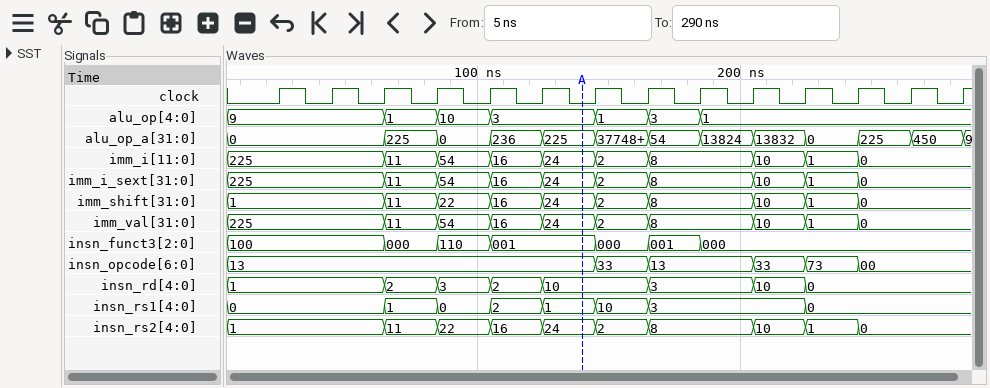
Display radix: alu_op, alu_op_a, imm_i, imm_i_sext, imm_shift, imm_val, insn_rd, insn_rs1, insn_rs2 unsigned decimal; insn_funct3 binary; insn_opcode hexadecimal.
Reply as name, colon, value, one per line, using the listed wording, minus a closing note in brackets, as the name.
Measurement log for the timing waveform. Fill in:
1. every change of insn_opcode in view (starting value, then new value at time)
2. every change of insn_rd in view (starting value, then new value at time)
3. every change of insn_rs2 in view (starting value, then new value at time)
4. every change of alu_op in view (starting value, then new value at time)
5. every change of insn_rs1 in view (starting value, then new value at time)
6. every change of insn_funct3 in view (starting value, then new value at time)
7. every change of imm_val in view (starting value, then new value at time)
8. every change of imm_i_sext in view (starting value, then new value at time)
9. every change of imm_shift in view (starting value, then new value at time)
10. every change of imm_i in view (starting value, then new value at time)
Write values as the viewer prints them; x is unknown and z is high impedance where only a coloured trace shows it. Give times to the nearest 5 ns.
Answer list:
every change of insn_opcode in view: 13, 33 at 145 ns, 13 at 165 ns, 33 at 205 ns, 73 at 225 ns, 00 at 245 ns
every change of insn_rd in view: 1, 2 at 65 ns, 3 at 85 ns, 2 at 105 ns, 10 at 125 ns, 3 at 165 ns, 10 at 205 ns, 0 at 225 ns
every change of insn_rs2 in view: 1, 11 at 65 ns, 22 at 85 ns, 16 at 105 ns, 24 at 125 ns, 2 at 145 ns, 8 at 165 ns, 10 at 205 ns, 1 at 225 ns, 0 at 245 ns
every change of alu_op in view: 9, 1 at 65 ns, 10 at 85 ns, 3 at 105 ns, 1 at 145 ns, 3 at 165 ns, 1 at 185 ns
every change of insn_rs1 in view: 0, 1 at 65 ns, 0 at 85 ns, 2 at 105 ns, 1 at 125 ns, 10 at 145 ns, 3 at 165 ns, 0 at 225 ns
every change of insn_funct3 in view: 100, 000 at 65 ns, 110 at 85 ns, 001 at 105 ns, 000 at 145 ns, 001 at 165 ns, 000 at 185 ns
every change of imm_val in view: 225, 11 at 65 ns, 54 at 85 ns, 16 at 105 ns, 24 at 125 ns, 2 at 145 ns, 8 at 165 ns, 10 at 205 ns, 1 at 225 ns, 0 at 245 ns
every change of imm_i_sext in view: 225, 11 at 65 ns, 54 at 85 ns, 16 at 105 ns, 24 at 125 ns, 2 at 145 ns, 8 at 165 ns, 10 at 205 ns, 1 at 225 ns, 0 at 245 ns
every change of imm_shift in view: 1, 11 at 65 ns, 22 at 85 ns, 16 at 105 ns, 24 at 125 ns, 2 at 145 ns, 8 at 165 ns, 10 at 205 ns, 1 at 225 ns, 0 at 245 ns
every change of imm_i in view: 225, 11 at 65 ns, 54 at 85 ns, 16 at 105 ns, 24 at 125 ns, 2 at 145 ns, 8 at 165 ns, 10 at 205 ns, 1 at 225 ns, 0 at 245 ns
